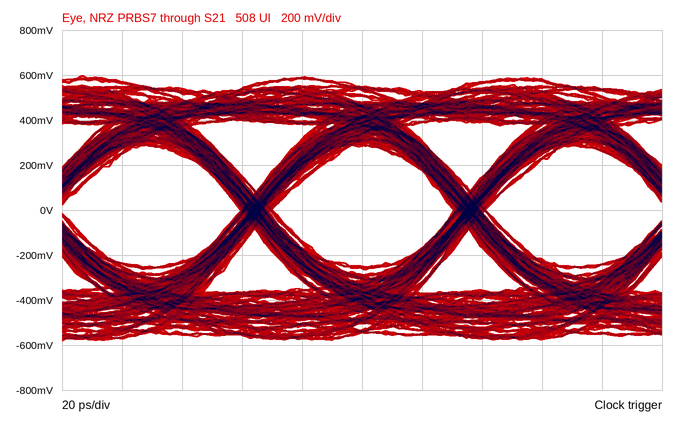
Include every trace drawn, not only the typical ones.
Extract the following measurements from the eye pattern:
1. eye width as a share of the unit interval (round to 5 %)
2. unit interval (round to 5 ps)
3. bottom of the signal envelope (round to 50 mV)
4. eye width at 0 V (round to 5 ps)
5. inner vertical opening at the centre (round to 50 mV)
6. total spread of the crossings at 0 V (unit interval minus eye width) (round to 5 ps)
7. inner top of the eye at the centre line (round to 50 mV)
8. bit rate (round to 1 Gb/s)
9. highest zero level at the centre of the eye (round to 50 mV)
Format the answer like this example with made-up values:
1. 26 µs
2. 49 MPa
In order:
1. 85 %
2. 70 ps
3. -600 mV
4. 60 ps
5. 550 mV
6. 10 ps
7. 300 mV
8. 14 Gb/s
9. -250 mV
